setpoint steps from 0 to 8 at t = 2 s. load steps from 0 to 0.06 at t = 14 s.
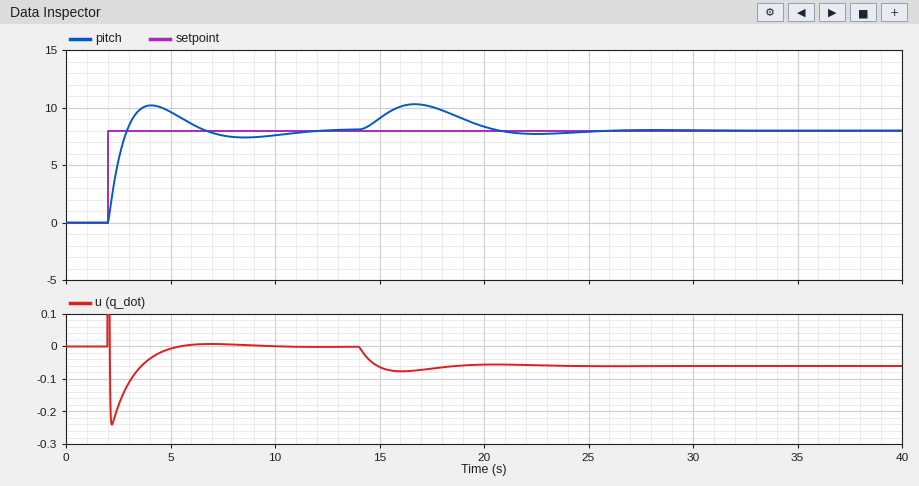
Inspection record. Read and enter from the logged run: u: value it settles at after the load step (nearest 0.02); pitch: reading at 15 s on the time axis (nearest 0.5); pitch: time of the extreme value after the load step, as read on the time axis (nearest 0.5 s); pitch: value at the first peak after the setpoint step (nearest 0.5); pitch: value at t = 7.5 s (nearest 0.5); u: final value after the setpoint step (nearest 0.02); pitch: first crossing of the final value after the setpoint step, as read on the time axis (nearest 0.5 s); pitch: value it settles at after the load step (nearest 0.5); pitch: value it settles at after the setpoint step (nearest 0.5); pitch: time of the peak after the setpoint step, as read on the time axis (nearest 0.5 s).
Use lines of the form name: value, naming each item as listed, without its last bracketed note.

u: value it settles at after the load step: -0.06
pitch: reading at 15 s on the time axis: 9.0
pitch: time of the extreme value after the load step, as read on the time axis: 16.5 s
pitch: value at the first peak after the setpoint step: 10.0
pitch: value at t = 7.5 s: 7.5
u: final value after the setpoint step: 0.00
pitch: first crossing of the final value after the setpoint step, as read on the time axis: 3.0 s
pitch: value it settles at after the load step: 8.0
pitch: value it settles at after the setpoint step: 8.0
pitch: time of the peak after the setpoint step, as read on the time axis: 4.0 s
